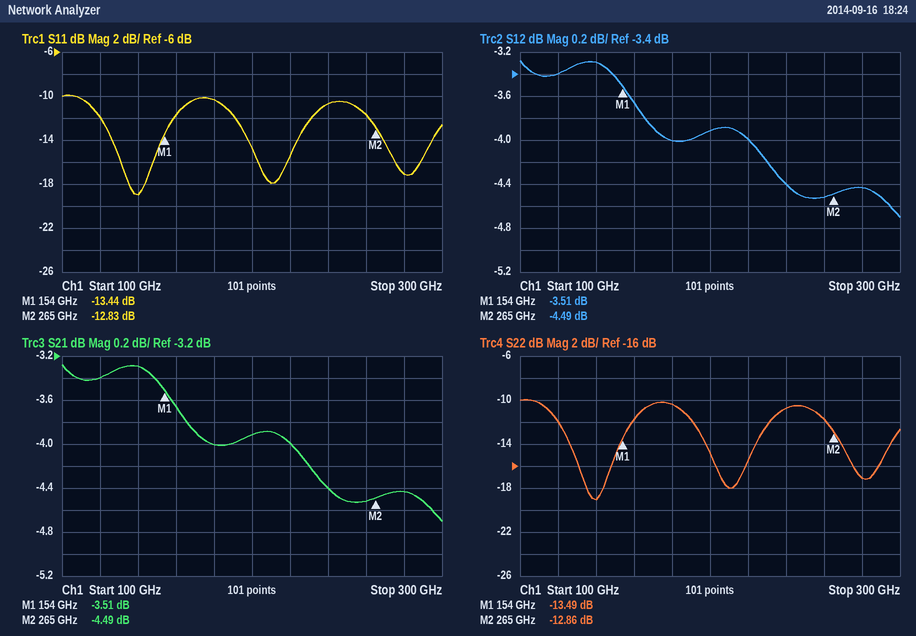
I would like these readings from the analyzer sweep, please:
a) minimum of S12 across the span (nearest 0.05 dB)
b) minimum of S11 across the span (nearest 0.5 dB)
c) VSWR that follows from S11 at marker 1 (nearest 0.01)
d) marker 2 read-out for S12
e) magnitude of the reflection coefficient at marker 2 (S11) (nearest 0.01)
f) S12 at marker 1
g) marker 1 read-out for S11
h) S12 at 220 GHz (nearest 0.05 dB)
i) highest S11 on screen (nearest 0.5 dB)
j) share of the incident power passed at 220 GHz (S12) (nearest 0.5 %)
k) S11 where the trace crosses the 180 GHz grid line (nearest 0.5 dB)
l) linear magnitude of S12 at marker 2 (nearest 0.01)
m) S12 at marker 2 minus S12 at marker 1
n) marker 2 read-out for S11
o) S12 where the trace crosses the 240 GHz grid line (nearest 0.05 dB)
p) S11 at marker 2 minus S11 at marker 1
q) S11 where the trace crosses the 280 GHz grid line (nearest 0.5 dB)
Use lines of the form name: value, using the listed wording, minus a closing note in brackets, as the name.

minimum of S12 across the span: -4.70 dB
minimum of S11 across the span: -19.0 dB
VSWR that follows from S11 at marker 1: 1.54
marker 2 read-out for S12: -4.49 dB
magnitude of the reflection coefficient at marker 2 (S11): 0.23
S12 at marker 1: -3.51 dB
marker 1 read-out for S11: -13.44 dB
S12 at 220 GHz: -4.00 dB
highest S11 on screen: -10.0 dB
share of the incident power passed at 220 GHz (S12): 40.0 %
S11 where the trace crosses the 180 GHz grid line: -10.5 dB
linear magnitude of S12 at marker 2: 0.60
S12 at marker 2 minus S12 at marker 1: -0.98 dB
marker 2 read-out for S11: -12.83 dB
S12 where the trace crosses the 240 GHz grid line: -4.40 dB
S11 at marker 2 minus S11 at marker 1: 0.61 dB
S11 where the trace crosses the 280 GHz grid line: -17.0 dB
